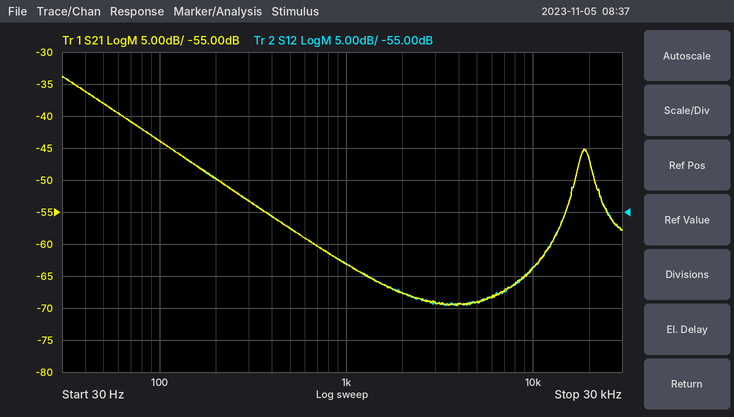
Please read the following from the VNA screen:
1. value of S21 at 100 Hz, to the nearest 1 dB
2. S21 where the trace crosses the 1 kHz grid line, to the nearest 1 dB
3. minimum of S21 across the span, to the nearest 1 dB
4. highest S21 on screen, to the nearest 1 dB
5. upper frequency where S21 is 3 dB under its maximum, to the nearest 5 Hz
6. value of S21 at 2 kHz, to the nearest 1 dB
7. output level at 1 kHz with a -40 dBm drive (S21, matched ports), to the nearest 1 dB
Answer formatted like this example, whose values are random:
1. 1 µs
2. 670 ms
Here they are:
1. -44 dB
2. -63 dB
3. -70 dB
4. -34 dB
5. 45 Hz
6. -68 dB
7. -103 dBm
